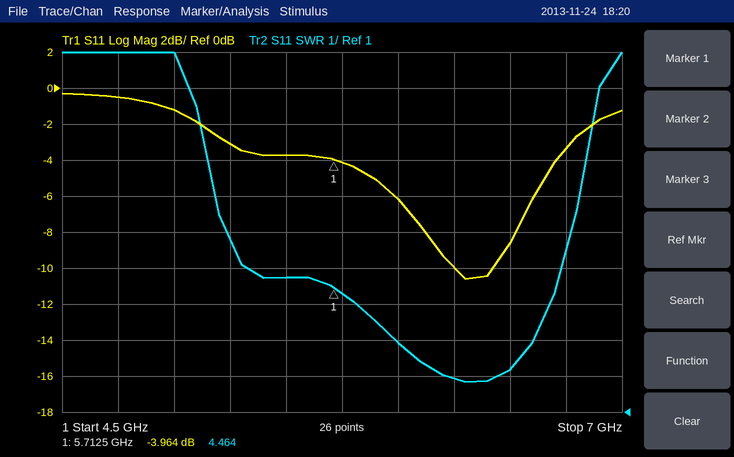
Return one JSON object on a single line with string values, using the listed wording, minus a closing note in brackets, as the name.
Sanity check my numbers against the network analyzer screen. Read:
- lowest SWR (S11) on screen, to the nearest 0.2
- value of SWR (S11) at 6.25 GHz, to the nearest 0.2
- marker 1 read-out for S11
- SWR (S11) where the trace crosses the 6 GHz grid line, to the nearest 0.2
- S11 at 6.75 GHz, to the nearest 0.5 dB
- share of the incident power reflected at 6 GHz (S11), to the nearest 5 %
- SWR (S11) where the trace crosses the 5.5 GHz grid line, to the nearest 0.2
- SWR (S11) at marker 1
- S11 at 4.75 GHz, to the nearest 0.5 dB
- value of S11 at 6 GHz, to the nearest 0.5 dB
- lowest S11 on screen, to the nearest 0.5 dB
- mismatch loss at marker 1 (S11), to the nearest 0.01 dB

{"lowest SWR (S11) on screen, to the nearest 0.2": "1.8", "value of SWR (S11) at 6.25 GHz, to the nearest 0.2": "2.0", "marker 1 read-out for S11": "-3.964 dB", "SWR (S11) where the trace crosses the 6 GHz grid line, to the nearest 0.2": "3.0", "S11 at 6.75 GHz, to the nearest 0.5 dB": "-3.5 dB", "share of the incident power reflected at 6 GHz (S11), to the nearest 5 %": "25 %", "SWR (S11) where the trace crosses the 5.5 GHz grid line, to the nearest 0.2": "4.8", "SWR (S11) at marker 1": "4.464", "S11 at 4.75 GHz, to the nearest 0.5 dB": "-0.5 dB", "value of S11 at 6 GHz, to the nearest 0.5 dB": "-6.0 dB", "lowest S11 on screen, to the nearest 0.5 dB": "-10.5 dB", "mismatch loss at marker 1 (S11), to the nearest 0.01 dB": "2.23 dB"}
